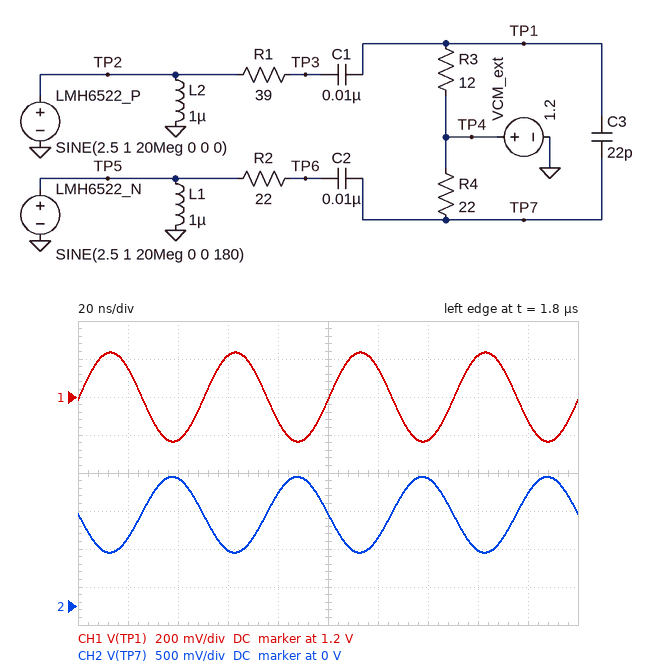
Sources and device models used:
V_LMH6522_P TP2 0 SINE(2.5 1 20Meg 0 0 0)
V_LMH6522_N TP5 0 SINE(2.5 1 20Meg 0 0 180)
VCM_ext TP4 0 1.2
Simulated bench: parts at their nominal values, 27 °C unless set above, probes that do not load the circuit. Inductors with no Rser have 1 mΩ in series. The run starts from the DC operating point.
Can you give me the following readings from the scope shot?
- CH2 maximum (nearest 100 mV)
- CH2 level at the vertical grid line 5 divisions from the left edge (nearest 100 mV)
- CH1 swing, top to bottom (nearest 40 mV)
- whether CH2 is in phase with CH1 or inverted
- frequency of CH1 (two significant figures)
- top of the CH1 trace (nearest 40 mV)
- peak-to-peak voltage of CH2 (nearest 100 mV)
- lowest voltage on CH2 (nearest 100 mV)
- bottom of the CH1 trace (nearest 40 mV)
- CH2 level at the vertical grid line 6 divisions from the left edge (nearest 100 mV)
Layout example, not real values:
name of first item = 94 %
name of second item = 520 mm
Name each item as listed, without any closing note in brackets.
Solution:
CH2 maximum = 1.7 V
CH2 level at the vertical grid line 5 divisions from the left edge = 1.2 V
CH1 swing, top to bottom = 480 mV
whether CH2 is in phase with CH1 or inverted = inverted
frequency of CH1 = 20 MHz
top of the CH1 trace = 1.44 V
peak-to-peak voltage of CH2 = 1.0 V
lowest voltage on CH2 = 700 mV
bottom of the CH1 trace = 960 mV
CH2 level at the vertical grid line 6 divisions from the left edge = 900 mV
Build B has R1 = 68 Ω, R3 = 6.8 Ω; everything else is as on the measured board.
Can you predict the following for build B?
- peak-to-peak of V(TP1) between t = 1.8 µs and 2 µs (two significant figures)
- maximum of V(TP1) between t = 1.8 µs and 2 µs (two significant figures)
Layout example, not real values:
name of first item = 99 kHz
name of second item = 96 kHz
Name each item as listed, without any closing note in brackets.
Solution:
peak-to-peak of V(TP1) between t = 1.8 µs and 2 µs = 180 mV
maximum of V(TP1) between t = 1.8 µs and 2 µs = 1.3 V
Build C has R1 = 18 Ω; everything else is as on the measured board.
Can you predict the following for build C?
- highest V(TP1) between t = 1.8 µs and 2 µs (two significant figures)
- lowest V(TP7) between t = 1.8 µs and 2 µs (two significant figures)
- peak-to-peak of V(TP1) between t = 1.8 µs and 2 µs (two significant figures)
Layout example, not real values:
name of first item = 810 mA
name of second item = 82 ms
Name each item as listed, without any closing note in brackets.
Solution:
highest V(TP1) between t = 1.8 µs and 2 µs = 1.6 V
lowest V(TP7) between t = 1.8 µs and 2 µs = 700 mV
peak-to-peak of V(TP1) between t = 1.8 µs and 2 µs = 800 mV
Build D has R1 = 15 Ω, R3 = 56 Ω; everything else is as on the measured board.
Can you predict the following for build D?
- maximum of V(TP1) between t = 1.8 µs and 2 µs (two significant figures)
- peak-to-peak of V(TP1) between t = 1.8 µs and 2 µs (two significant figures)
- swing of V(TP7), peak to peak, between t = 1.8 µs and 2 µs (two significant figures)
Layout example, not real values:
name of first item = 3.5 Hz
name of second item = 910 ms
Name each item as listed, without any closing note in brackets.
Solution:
maximum of V(TP1) between t = 1.8 µs and 2 µs = 2.0 V
peak-to-peak of V(TP1) between t = 1.8 µs and 2 µs = 1.6 V
swing of V(TP7), peak to peak, between t = 1.8 µs and 2 µs = 1.0 V
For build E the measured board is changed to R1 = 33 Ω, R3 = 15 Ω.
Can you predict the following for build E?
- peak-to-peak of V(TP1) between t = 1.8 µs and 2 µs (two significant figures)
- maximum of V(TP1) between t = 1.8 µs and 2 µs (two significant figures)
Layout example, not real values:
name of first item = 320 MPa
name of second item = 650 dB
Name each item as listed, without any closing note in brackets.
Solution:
peak-to-peak of V(TP1) between t = 1.8 µs and 2 µs = 620 mV
maximum of V(TP1) between t = 1.8 µs and 2 µs = 1.5 V
